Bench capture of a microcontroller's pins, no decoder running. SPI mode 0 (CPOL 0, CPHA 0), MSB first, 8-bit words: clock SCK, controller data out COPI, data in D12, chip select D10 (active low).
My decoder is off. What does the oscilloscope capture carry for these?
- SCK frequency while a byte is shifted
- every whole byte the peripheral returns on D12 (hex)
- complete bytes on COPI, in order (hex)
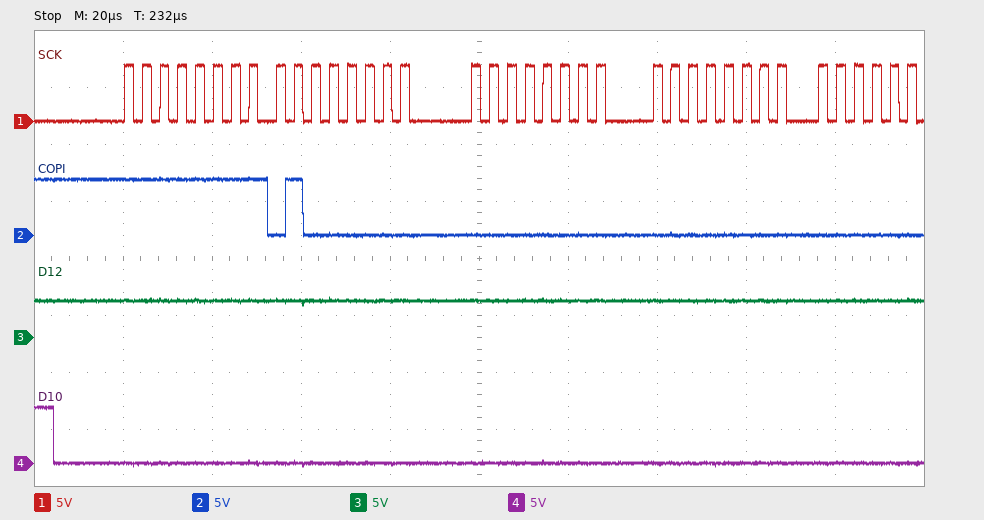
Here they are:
250 kHz
FF FF FF FF
FF 40 00 00
